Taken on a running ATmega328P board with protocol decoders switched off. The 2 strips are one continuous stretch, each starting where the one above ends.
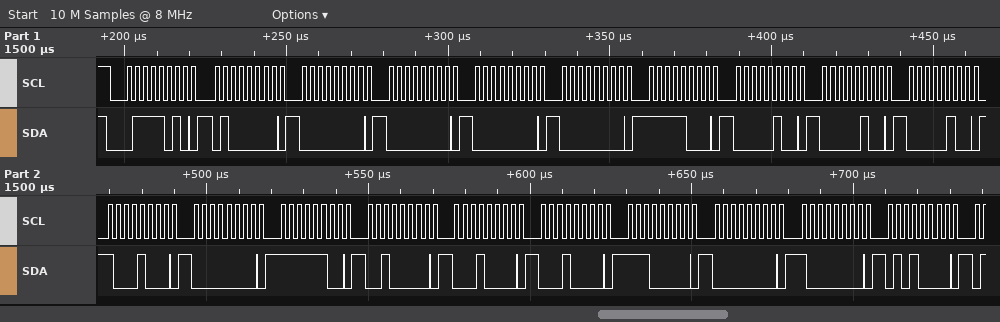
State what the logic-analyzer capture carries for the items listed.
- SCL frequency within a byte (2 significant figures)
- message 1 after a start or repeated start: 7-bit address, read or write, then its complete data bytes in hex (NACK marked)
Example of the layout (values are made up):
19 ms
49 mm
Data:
400 kHz
0x3D write: 40 00 00 00 00 F8 04 04 04 88 00 FC 20 10 10 E0 00 80 50
